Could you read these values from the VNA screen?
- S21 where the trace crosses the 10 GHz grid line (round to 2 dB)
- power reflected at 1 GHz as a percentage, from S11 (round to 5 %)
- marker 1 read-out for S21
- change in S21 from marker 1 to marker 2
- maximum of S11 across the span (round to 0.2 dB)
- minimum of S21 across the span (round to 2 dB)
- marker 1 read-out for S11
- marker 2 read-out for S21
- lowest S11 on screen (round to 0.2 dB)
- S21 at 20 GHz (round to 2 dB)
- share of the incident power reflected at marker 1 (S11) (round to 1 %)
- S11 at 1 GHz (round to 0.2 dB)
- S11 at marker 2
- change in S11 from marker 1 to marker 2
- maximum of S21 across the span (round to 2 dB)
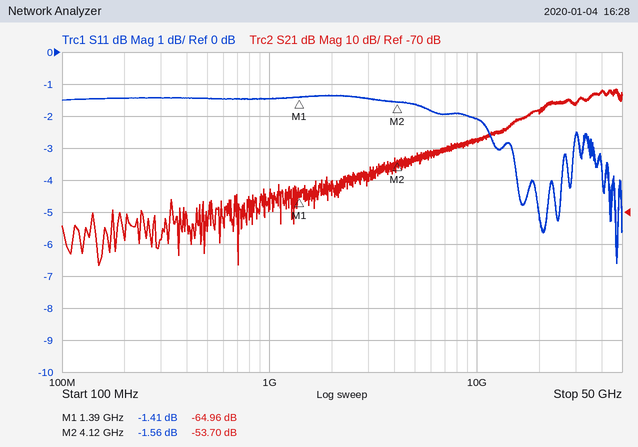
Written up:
-48 dB
70 %
-64.96 dB
11.26 dB
-1.4 dB
-86 dB
-1.41 dB
-53.70 dB
-6.6 dB
-38 dB
72 %
-1.4 dB
-1.56 dB
-0.15 dB
-32 dB
